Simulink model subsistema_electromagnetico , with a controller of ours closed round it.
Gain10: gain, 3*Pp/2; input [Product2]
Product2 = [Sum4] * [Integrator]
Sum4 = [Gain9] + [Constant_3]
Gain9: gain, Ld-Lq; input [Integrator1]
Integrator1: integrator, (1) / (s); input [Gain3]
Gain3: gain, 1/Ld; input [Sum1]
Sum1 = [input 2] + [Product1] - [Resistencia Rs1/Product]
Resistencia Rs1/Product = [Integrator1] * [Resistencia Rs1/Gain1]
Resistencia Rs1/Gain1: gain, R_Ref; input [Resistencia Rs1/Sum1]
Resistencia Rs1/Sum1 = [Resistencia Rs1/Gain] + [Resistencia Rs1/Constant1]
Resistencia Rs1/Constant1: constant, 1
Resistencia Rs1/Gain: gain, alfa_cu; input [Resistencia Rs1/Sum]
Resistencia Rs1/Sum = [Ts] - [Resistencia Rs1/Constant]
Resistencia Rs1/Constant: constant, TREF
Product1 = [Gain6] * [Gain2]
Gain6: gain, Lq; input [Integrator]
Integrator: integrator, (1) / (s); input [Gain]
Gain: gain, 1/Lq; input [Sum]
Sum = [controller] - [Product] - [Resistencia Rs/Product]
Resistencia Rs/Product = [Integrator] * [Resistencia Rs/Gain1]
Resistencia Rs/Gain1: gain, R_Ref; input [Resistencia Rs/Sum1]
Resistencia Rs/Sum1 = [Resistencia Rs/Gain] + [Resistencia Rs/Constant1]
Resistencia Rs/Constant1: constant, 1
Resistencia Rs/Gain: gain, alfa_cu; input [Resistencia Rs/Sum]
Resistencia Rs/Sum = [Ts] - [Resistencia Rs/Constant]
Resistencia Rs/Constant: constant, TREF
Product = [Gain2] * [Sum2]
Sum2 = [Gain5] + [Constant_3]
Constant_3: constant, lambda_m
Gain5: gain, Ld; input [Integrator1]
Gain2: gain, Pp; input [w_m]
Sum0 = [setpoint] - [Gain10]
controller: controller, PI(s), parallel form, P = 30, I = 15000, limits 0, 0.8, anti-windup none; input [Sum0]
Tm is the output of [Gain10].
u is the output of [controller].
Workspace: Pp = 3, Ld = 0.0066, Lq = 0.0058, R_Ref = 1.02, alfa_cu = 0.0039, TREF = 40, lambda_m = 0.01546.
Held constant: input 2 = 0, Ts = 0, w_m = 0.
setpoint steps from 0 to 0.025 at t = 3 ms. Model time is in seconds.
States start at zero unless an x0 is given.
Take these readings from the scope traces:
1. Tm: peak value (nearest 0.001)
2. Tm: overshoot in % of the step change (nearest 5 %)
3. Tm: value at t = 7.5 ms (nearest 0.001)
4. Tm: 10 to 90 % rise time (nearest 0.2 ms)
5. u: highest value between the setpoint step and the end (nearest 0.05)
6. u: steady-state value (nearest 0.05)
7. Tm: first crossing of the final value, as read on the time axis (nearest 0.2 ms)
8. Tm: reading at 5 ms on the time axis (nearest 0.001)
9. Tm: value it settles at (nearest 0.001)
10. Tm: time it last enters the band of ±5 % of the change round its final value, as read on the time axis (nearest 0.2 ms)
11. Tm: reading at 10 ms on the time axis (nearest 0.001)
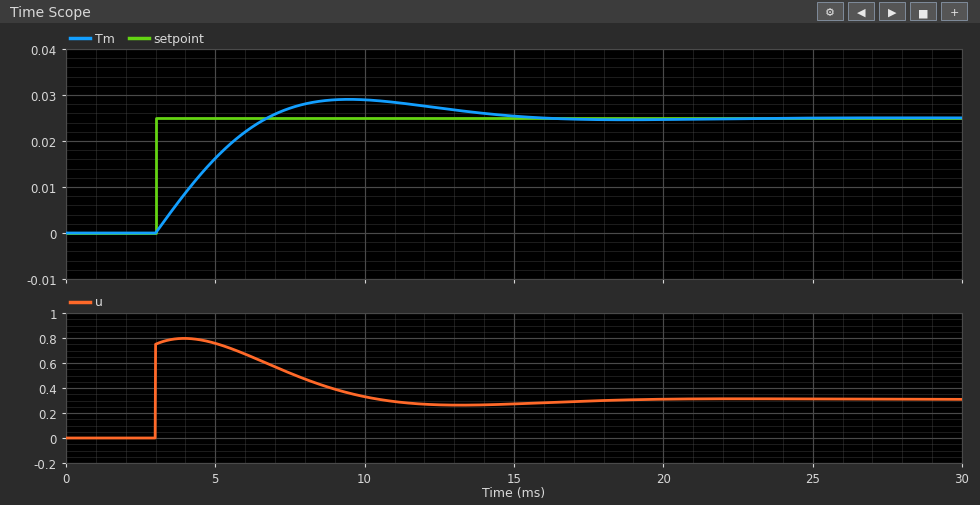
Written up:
0.029
15 %
0.027
2.8 ms
0.80
0.30
6.8 ms
0.016
0.025
13.6 ms
0.029
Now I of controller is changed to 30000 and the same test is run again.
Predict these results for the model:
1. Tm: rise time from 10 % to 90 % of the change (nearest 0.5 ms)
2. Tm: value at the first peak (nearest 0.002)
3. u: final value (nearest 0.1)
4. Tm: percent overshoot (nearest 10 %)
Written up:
2.5 ms
0.034
0.3
40 %
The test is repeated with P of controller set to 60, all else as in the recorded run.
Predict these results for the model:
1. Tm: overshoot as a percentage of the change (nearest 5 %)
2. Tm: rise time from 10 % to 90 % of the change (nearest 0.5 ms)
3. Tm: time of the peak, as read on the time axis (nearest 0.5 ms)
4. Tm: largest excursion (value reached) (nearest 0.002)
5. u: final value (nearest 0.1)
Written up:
10 %
2.5 ms
9.0 ms
0.028
0.3
